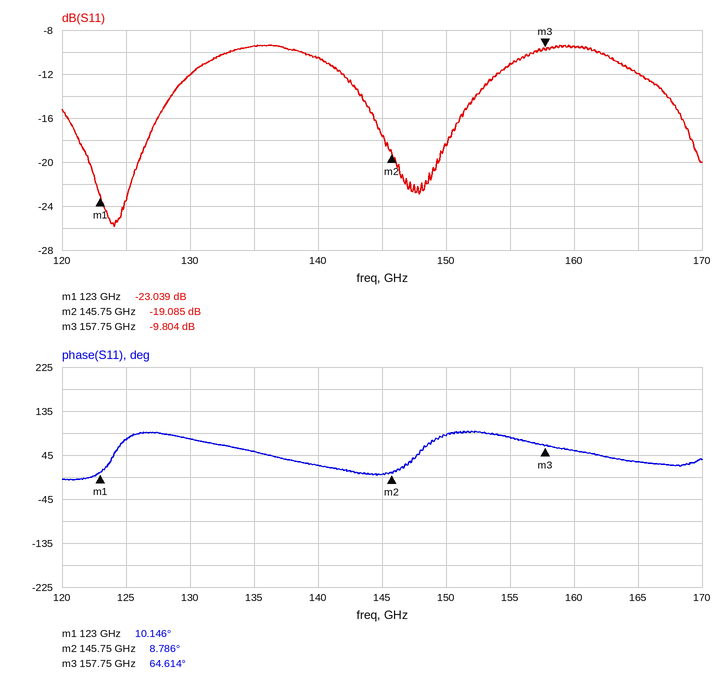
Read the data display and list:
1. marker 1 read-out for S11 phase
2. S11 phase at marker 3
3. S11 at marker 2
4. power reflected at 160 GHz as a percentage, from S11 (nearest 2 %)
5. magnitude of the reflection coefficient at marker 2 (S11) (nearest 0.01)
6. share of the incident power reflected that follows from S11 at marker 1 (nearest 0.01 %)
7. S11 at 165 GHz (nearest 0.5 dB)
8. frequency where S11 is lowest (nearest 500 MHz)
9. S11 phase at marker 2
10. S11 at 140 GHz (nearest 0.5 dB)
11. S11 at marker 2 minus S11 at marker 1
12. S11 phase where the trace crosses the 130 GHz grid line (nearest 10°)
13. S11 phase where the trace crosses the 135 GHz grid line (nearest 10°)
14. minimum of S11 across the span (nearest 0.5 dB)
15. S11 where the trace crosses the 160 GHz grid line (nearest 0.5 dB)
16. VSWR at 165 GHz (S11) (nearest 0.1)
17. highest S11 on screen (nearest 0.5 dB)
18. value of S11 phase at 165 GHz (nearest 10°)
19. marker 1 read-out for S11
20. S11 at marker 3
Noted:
10.146°
64.614°
-19.085 dB
12 %
0.11
0.50 %
-12.0 dB
124.0 GHz
8.786°
-10.5 dB
3.954 dB
80°
50°
-26.0 dB
-9.5 dB
1.7
-9.5 dB
30°
-23.039 dB
-9.804 dB
